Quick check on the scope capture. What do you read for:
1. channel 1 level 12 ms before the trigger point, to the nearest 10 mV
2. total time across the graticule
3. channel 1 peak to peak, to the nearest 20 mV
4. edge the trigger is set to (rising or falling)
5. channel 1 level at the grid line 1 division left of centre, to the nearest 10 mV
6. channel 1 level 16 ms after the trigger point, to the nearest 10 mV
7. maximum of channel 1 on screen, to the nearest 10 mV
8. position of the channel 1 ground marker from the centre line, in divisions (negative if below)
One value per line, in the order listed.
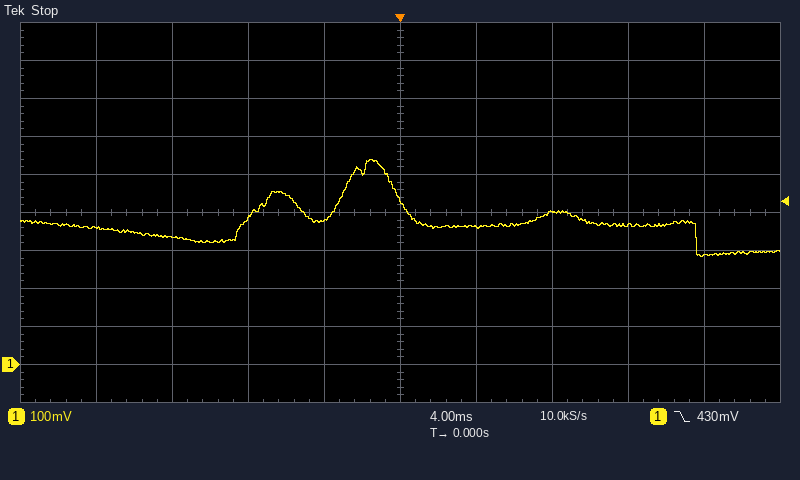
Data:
340 mV
40 ms
260 mV
falling
380 mV
290 mV
540 mV
-4.0 div
